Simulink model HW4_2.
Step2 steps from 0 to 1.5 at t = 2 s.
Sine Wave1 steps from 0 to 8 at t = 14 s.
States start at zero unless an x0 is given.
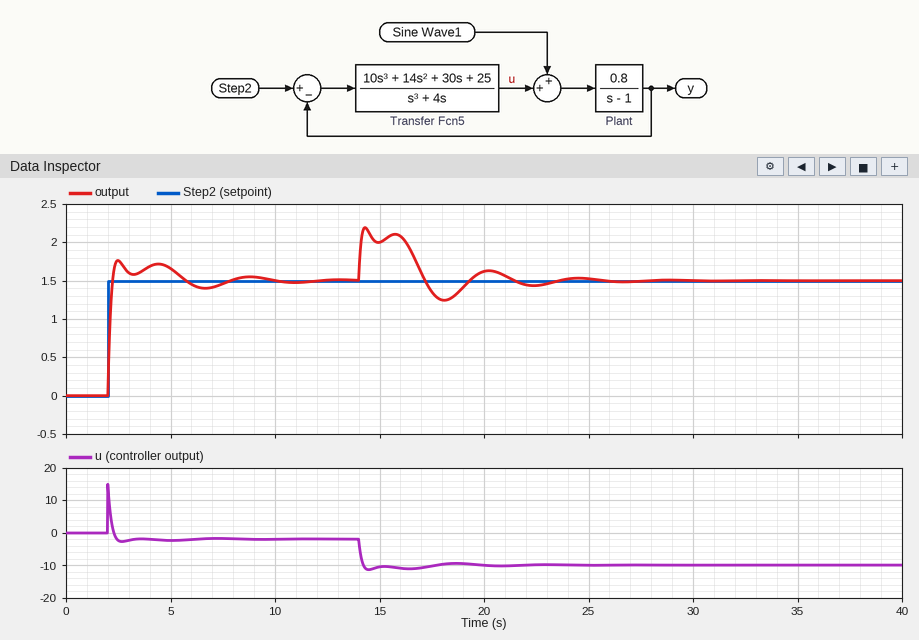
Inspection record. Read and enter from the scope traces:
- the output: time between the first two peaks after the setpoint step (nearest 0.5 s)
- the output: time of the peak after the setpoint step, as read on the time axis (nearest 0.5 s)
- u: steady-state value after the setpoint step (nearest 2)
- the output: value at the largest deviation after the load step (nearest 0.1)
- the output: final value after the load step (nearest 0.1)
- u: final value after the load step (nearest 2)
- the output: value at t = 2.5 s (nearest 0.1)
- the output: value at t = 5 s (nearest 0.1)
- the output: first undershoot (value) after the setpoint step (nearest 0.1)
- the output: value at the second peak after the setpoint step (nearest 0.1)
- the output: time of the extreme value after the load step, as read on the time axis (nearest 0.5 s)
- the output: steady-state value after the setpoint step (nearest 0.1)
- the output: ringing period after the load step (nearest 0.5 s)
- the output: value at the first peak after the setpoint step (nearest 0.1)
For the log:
2.0 s
2.5 s
-2
2.2
1.5
-10
1.8
1.7
1.6
1.7
14.5 s
1.5
1.5 s
1.8
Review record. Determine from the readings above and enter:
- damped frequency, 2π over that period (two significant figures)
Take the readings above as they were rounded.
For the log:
3.1 rad/s
